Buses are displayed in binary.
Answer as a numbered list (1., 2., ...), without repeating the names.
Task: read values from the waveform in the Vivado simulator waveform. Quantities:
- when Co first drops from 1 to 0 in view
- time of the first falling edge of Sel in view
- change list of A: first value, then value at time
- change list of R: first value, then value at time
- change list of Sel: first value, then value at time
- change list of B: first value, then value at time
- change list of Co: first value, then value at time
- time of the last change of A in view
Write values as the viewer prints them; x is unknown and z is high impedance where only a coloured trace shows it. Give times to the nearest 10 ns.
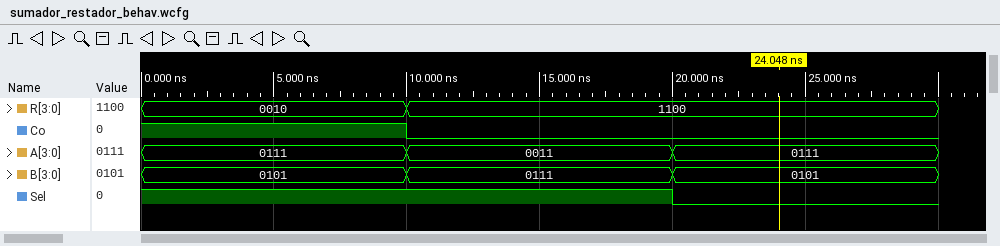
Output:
1. 10 ns
2. 20 ns
3. 0111, 0011 at 10 ns, 0111 at 20 ns
4. 0010, 1100 at 10 ns
5. 1, 0 at 20 ns
6. 0101, 0111 at 10 ns, 0101 at 20 ns
7. 1, 0 at 10 ns
8. 20 ns
